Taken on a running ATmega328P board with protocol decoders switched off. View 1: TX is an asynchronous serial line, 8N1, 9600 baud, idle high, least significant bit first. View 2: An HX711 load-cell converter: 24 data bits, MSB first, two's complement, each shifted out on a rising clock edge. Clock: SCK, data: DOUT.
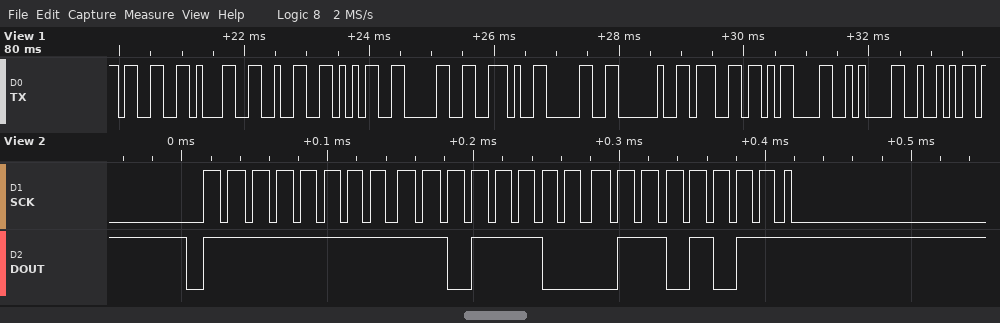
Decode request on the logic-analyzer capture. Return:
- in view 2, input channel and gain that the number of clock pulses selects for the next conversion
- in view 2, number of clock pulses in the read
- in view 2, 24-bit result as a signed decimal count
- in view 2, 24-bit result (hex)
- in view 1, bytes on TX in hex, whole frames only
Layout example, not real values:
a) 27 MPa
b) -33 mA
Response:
a) channel A, gain 128
b) 25
c) -9109
d) 0xFFDC6B
e) 33 31 32 35 30 2E 30 20 67 0D 0A 52
